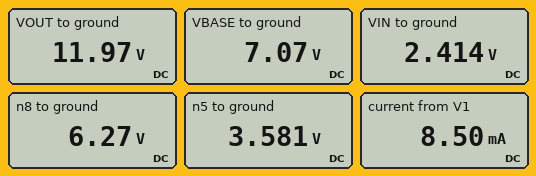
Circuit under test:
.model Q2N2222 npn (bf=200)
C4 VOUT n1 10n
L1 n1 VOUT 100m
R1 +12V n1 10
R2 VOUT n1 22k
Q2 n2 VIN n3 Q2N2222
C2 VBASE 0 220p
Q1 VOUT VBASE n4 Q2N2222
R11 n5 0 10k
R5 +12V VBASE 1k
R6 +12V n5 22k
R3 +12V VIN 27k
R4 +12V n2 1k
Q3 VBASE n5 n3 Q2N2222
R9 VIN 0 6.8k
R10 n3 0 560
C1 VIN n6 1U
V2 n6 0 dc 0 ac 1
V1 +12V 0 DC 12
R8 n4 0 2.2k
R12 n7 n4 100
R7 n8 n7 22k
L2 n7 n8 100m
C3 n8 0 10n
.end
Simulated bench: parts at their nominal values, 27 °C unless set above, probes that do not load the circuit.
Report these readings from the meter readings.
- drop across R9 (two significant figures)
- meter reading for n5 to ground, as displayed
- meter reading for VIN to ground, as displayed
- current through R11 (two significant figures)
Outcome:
2.4 V
3.581 V
2.414 V
360 µA
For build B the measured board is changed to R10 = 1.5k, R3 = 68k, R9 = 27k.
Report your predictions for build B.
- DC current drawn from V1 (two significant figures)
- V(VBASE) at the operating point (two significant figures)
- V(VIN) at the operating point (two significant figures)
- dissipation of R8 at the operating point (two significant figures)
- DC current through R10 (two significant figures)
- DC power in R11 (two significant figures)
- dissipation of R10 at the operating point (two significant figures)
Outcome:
6.6 mA
10 V
3.4 V
39 mW
1.9 mA
1.4 mW
5.6 mW
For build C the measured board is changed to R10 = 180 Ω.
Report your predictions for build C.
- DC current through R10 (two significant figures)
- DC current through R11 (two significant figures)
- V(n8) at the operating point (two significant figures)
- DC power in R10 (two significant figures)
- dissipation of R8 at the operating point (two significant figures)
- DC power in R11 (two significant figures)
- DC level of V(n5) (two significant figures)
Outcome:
10 mA
270 µA
1.2 V
19 mW
650 µW
710 µW
2.7 V
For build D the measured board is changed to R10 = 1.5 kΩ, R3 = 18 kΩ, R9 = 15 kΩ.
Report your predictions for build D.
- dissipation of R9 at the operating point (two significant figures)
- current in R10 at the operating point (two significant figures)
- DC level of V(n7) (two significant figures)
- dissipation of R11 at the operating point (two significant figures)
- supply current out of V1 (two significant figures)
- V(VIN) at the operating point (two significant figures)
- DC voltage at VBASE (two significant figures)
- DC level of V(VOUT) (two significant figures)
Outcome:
1.9 mW
3.0 mA
11 V
1.4 mW
8.8 mA
5.3 V
12 V
12 V
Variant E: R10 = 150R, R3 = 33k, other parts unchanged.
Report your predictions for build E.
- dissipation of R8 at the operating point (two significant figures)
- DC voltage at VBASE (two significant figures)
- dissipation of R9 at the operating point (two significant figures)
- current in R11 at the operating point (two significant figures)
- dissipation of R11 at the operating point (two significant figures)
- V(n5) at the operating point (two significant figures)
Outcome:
400 µW
1.7 V
620 µW
240 µA
580 µW
2.4 V
